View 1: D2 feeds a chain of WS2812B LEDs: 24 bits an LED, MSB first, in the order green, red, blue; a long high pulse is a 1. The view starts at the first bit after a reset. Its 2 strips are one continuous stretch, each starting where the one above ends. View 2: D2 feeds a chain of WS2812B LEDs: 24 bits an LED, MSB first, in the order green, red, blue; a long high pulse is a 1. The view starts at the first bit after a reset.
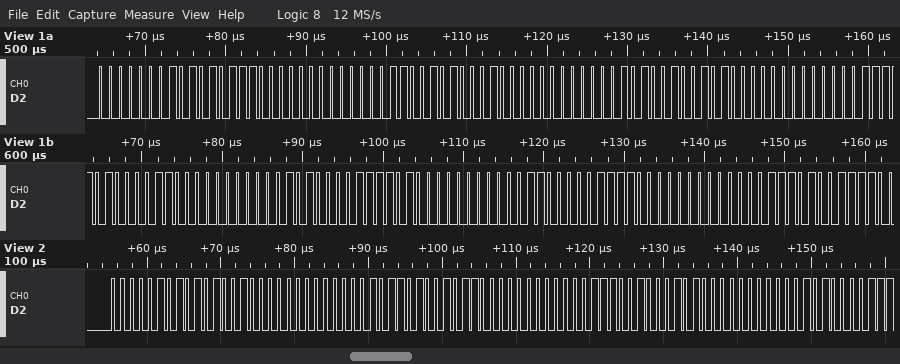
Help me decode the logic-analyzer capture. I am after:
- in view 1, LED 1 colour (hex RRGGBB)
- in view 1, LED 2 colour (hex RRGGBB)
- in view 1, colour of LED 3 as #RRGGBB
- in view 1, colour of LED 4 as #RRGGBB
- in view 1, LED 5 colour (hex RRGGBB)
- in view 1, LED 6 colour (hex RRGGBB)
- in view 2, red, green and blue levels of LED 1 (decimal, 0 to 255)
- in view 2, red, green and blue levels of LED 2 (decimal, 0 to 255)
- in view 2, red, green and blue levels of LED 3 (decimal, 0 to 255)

#570100
#510600
#4A0A00
#430F00
#3D1400
#3C1800
82, 5, 0
75, 11, 0
69, 14, 0
